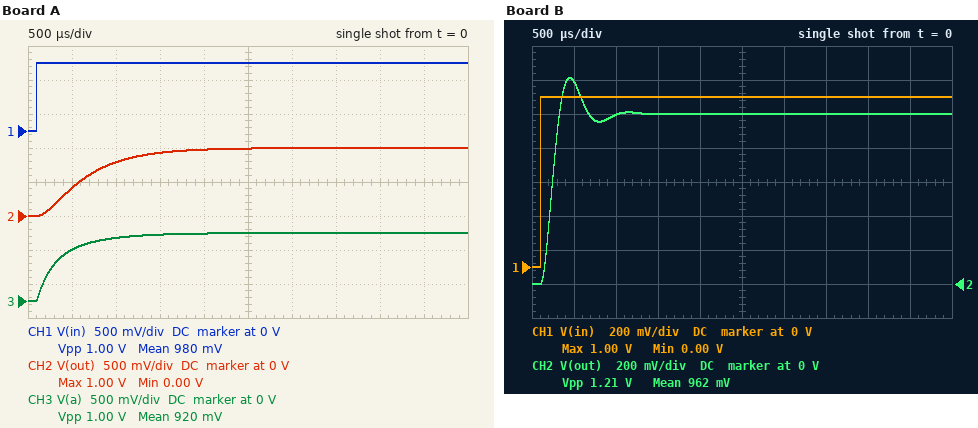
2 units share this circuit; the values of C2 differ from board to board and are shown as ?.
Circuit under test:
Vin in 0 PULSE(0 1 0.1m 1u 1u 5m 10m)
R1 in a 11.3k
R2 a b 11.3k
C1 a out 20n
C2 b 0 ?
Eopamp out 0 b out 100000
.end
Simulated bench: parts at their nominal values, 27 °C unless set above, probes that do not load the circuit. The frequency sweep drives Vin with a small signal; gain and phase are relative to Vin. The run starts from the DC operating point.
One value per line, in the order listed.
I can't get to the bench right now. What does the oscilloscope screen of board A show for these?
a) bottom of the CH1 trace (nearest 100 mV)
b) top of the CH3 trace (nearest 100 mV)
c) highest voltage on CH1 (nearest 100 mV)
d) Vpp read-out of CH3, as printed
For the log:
0 V
1.0 V
1.0 V
1.00 V
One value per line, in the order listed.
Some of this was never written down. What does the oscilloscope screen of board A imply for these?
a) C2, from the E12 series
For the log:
27 nF
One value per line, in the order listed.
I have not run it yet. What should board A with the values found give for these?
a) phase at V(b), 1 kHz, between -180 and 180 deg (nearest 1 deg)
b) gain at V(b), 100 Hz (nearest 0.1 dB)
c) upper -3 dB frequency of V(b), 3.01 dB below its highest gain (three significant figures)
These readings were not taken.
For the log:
-114 deg
-0.4 dB
316 Hz
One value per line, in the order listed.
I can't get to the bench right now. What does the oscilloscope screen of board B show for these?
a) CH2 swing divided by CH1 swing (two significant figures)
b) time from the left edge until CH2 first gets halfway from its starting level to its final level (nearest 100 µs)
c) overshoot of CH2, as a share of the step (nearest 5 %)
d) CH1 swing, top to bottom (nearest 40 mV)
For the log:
1.2
200 µs
20 %
1.00 V
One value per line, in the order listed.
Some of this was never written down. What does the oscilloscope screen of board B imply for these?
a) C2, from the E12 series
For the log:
3.9 nF
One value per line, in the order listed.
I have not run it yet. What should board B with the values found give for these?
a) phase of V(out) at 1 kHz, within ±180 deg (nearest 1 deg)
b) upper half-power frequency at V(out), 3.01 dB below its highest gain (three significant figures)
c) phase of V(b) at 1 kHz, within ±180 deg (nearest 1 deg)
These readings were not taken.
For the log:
-42 deg
1.89 kHz
-42 deg
